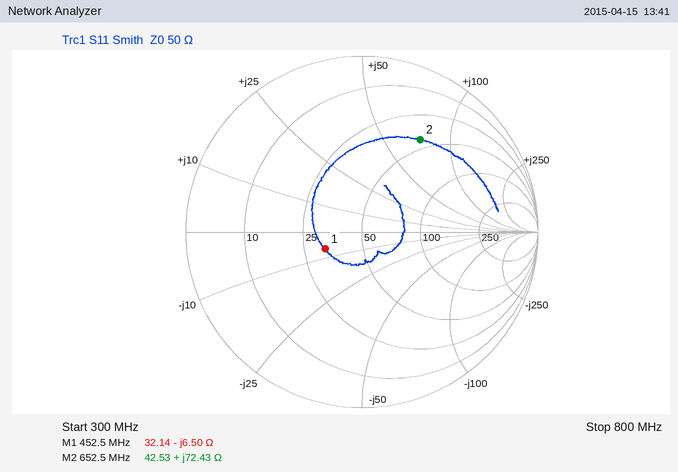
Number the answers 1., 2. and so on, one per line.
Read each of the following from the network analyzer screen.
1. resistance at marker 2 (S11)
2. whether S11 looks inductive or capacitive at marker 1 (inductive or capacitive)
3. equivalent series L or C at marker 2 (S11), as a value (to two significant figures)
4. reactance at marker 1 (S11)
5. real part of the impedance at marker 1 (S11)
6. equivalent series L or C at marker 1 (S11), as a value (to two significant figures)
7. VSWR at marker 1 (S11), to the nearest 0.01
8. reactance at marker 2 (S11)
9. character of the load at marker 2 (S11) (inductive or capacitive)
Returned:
1. 42.53 Ω
2. capacitive
3. 18 nH
4. -6.50 Ω
5. 32.14 Ω
6. 54 pF
7. 1.60
8. +72.43 Ω
9. inductive
